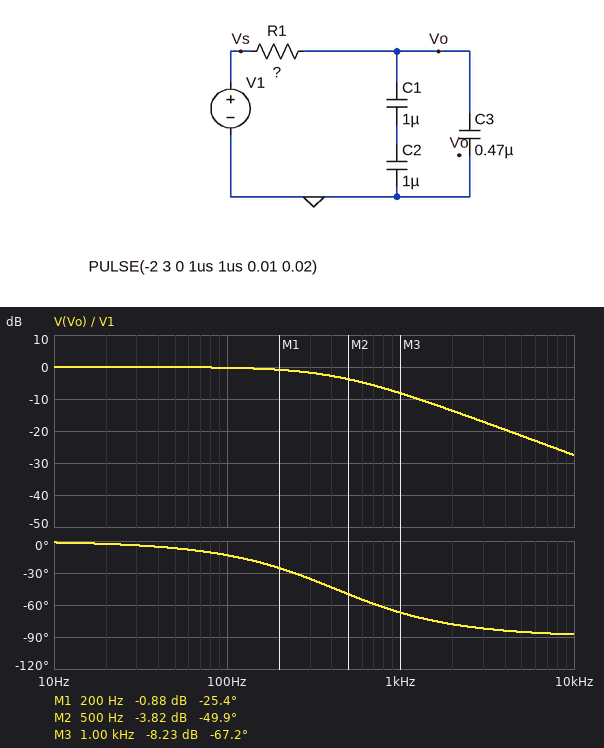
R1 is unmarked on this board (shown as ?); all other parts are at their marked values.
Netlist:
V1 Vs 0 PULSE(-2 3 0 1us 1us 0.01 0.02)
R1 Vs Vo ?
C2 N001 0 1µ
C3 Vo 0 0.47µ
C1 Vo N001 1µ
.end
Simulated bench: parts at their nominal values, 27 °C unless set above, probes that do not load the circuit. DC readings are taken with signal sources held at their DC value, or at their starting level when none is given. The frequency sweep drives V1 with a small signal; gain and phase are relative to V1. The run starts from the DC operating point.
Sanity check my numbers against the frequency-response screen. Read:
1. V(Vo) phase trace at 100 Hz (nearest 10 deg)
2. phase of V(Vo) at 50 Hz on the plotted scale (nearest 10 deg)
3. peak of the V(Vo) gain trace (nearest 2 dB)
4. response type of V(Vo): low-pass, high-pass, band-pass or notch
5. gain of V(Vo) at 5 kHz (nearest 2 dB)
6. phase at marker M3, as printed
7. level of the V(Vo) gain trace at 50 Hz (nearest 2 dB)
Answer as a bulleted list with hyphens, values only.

- -10 deg
- -10 deg
- 0 dB
- low-pass
- -22 dB
- -67.2 deg
- 0 dB
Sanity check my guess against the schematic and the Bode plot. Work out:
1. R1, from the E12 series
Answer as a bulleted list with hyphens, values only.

- 390 Ω
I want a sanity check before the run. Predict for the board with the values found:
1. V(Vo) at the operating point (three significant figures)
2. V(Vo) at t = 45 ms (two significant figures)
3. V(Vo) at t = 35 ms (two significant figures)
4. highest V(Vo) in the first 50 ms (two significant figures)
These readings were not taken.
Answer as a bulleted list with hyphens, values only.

- -2.00 V
- 3.0 V
- -2.0 V
- 3.0 V
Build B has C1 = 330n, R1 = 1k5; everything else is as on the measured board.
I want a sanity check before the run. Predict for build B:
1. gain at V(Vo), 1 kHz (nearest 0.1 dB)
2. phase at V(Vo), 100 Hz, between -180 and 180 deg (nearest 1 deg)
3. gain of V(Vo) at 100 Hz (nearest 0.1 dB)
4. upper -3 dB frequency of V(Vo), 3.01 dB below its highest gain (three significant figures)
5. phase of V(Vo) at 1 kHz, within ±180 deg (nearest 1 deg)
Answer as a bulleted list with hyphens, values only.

- -16.7 dB
- -34 deg
- -1.6 dB
- 148 Hz
- -82 deg
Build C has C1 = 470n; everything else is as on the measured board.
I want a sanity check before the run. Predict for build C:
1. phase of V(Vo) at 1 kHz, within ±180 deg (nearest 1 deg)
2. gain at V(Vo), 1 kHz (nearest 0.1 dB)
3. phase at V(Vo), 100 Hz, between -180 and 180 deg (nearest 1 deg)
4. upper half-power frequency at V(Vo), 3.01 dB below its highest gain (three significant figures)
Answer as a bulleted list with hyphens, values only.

- -63 deg
- -6.8 dB
- -11 deg
- 517 Hz
